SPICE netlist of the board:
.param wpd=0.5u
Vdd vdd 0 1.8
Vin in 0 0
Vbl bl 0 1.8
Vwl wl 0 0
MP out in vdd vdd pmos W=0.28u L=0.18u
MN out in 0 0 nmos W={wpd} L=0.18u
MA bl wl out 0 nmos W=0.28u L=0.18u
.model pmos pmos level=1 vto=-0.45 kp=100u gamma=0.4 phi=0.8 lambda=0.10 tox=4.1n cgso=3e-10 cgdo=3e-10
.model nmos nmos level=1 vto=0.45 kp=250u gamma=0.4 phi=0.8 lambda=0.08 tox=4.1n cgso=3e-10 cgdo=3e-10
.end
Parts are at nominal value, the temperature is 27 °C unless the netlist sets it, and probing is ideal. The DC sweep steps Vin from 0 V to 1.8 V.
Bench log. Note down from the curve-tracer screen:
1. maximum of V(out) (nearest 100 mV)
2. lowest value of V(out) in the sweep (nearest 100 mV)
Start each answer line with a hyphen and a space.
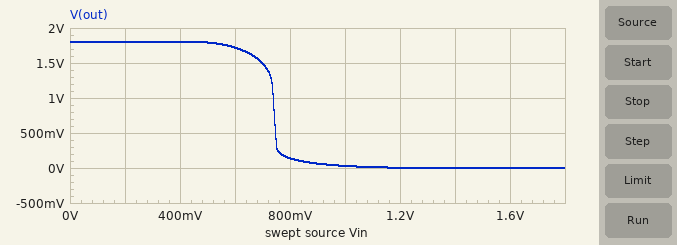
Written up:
- 1.8 V
- 0 V
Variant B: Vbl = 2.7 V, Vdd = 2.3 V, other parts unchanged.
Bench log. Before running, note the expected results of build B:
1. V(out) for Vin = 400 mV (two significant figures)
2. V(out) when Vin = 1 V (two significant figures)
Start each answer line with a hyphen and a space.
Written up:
- 2.3 V
- 220 mV
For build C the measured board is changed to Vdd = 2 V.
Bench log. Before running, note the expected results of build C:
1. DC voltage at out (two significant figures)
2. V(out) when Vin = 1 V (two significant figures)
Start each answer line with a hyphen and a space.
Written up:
- 2.0 V
- 79 mV
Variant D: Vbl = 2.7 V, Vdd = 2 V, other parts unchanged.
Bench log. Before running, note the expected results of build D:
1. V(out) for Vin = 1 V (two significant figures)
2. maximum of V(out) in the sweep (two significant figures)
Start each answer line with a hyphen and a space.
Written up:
- 79 mV
- 2.0 V
